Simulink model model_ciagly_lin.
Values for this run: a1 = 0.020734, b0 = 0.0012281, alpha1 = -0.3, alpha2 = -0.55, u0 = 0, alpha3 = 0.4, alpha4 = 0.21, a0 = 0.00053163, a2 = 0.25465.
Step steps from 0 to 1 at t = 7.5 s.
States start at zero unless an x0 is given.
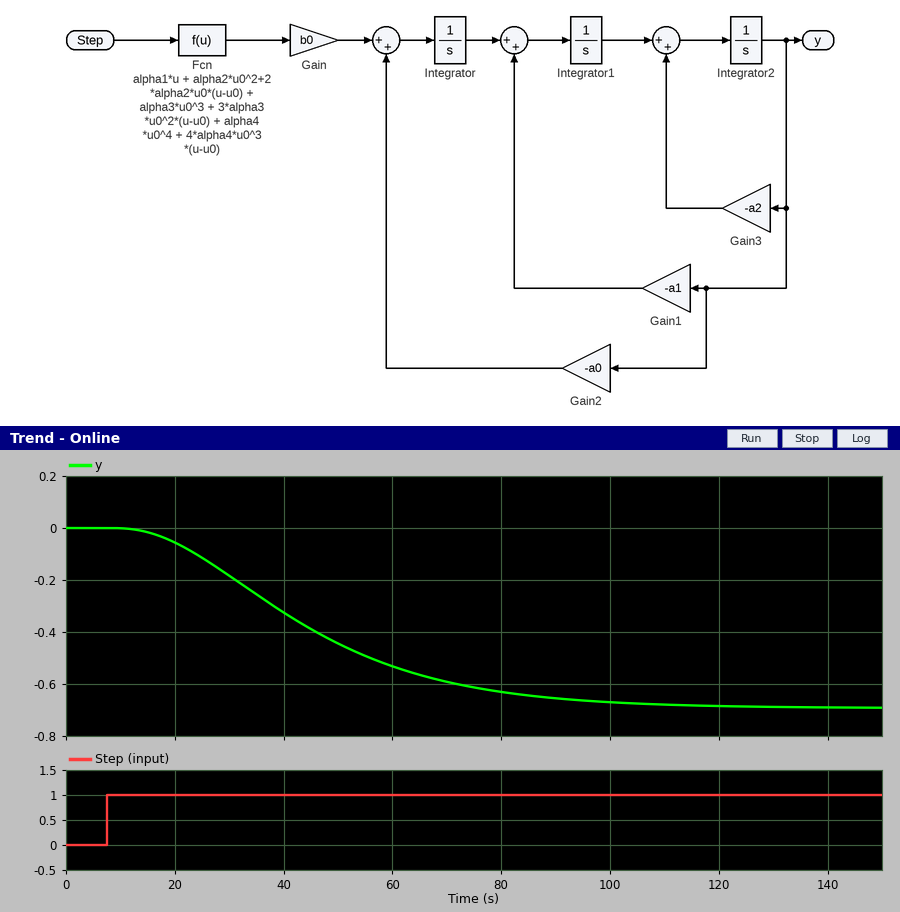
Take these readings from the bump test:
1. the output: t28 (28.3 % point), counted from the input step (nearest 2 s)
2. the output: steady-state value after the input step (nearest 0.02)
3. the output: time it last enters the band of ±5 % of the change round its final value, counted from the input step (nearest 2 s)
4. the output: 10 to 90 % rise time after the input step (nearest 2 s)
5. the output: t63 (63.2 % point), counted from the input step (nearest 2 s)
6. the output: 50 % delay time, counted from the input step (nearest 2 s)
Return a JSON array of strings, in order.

["24 s", "-0.70", "84 s", "56 s", "42 s", "34 s"]
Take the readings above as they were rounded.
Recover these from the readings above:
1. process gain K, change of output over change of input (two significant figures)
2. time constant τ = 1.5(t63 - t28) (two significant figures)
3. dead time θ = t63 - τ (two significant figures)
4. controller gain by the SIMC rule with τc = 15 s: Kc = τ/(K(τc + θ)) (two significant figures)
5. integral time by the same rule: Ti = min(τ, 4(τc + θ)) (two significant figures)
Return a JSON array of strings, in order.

["-0.70", "27 s", "15 s", "-1.3", "27 s"]
